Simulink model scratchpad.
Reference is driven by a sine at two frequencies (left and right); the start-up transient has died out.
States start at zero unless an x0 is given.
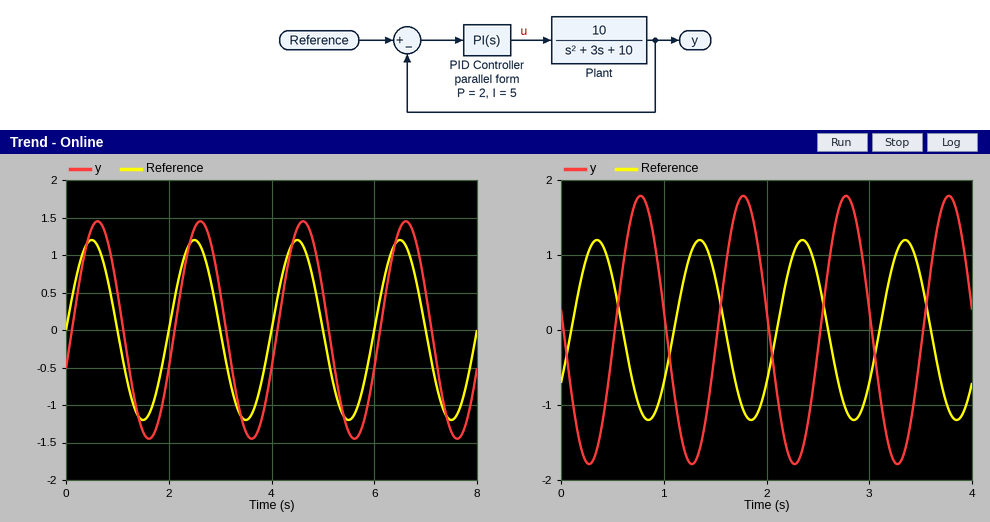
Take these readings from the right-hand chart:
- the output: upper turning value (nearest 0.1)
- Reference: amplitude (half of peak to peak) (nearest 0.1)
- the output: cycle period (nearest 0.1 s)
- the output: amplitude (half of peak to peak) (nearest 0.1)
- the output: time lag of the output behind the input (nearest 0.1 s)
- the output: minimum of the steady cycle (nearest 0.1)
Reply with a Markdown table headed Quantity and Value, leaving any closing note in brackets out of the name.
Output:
| Quantity | Value |
|---|---|
| the output: upper turning value | 1.8 |
| Reference: amplitude (half of peak to peak) | 1.2 |
| the output: cycle period | 1.0 s |
| the output: amplitude (half of peak to peak) | 1.8 |
| the output: time lag of the output behind the input | 0.4 s |
| the output: minimum of the steady cycle | -1.8 |
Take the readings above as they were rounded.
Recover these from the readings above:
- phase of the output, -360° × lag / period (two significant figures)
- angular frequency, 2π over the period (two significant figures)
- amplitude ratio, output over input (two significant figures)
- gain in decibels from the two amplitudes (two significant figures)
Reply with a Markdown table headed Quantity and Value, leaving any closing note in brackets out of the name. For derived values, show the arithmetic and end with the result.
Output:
| Quantity | Value |
|---|---|
| phase of the output, -360° × lag / period | -360 × 0.4 / 1 = -140° |
| angular frequency, 2π over the period | 2π / 1 = 6.3 rad/s |
| amplitude ratio, output over input | 1.8 / 1.2 = 1.5 |
| gain in decibels from the two amplitudes | 20 log10(1.8 / 1.2) = 3.5 dB |
